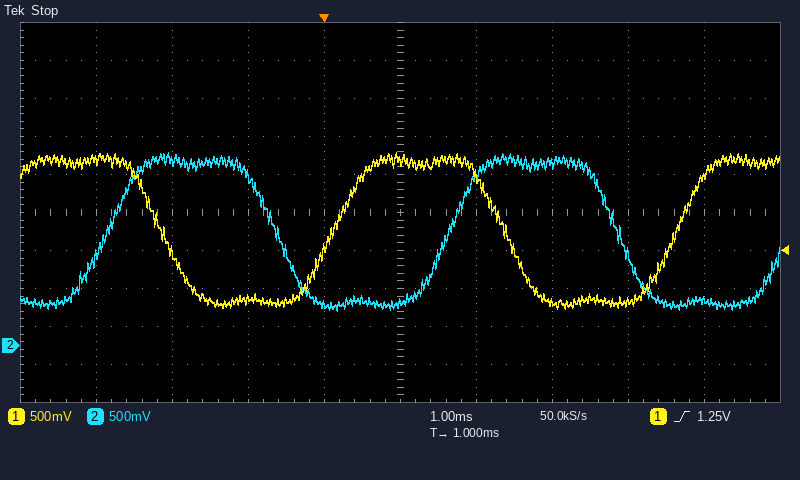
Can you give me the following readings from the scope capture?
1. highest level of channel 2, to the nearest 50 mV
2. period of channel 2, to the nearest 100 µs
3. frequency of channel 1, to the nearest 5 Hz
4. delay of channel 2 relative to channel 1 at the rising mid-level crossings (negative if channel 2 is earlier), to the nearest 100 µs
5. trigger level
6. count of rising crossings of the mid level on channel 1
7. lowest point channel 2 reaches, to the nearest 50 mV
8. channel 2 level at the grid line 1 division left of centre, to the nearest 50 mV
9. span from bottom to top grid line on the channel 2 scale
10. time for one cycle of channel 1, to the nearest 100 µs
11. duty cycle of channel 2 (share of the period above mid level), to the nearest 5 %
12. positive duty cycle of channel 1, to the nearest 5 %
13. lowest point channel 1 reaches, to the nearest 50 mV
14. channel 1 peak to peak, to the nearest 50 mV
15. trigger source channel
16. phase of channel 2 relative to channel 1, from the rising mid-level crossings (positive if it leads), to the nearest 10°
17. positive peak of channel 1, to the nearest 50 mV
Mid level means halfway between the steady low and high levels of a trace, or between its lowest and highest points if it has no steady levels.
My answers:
2.55 V
4.5 ms
220 Hz
+1.5 ms
1.25 V
2
450 mV
550 mV
5 V
4.5 ms
50 %
50 %
500 mV
2.05 V
channel 1
-120°
2.55 V
